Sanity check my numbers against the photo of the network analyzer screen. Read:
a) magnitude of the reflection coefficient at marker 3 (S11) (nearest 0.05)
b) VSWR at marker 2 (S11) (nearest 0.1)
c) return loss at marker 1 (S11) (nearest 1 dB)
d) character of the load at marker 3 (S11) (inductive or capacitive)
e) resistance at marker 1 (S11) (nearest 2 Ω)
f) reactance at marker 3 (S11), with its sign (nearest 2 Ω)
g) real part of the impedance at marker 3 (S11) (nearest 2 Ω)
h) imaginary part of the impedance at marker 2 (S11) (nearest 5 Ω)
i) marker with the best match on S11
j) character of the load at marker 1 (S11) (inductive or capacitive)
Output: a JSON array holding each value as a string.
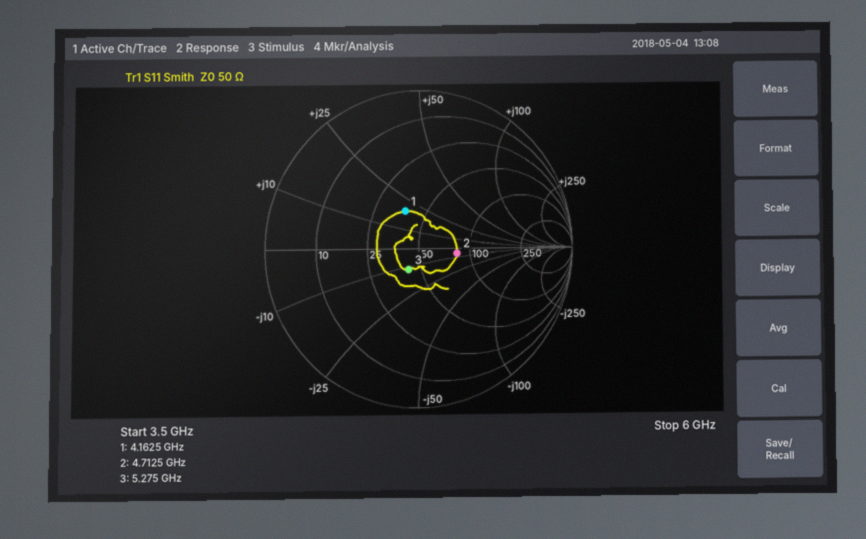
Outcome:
["0.15", "1.7", "12 dB", "capacitive", "38 Ω", "-12 Ω", "42 Ω", "-5 Ω", "marker 3", "inductive"]
